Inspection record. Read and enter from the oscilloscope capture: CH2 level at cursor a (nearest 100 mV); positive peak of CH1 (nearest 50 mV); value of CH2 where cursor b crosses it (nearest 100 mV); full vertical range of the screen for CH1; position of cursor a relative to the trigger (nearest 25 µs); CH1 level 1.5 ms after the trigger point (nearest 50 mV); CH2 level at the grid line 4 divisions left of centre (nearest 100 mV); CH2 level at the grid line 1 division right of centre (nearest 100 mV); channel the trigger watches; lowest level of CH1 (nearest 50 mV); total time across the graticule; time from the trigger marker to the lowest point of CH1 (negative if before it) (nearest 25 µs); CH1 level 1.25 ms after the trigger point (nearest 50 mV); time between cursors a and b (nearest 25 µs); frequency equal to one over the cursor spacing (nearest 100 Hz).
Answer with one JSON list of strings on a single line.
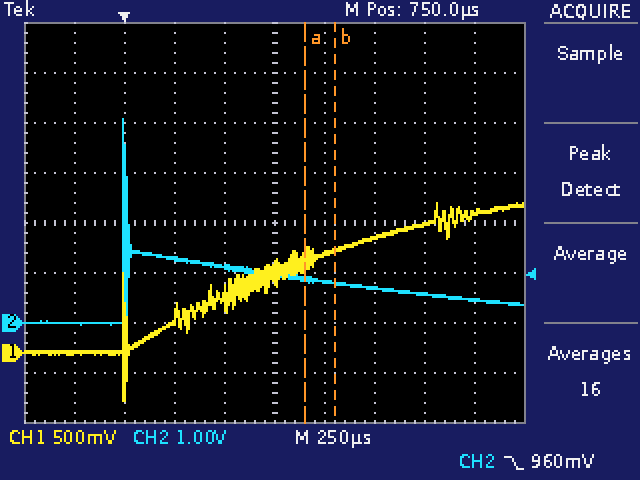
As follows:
["900 mV", "1.50 V", "800 mV", "4 V", "+900 µs", "1.30 V", "0.0 V", "800 mV", "CH2", "-500 mV", "2.5 ms", "0 µs", "1.15 V", "150 µs", "6.7 kHz"]
